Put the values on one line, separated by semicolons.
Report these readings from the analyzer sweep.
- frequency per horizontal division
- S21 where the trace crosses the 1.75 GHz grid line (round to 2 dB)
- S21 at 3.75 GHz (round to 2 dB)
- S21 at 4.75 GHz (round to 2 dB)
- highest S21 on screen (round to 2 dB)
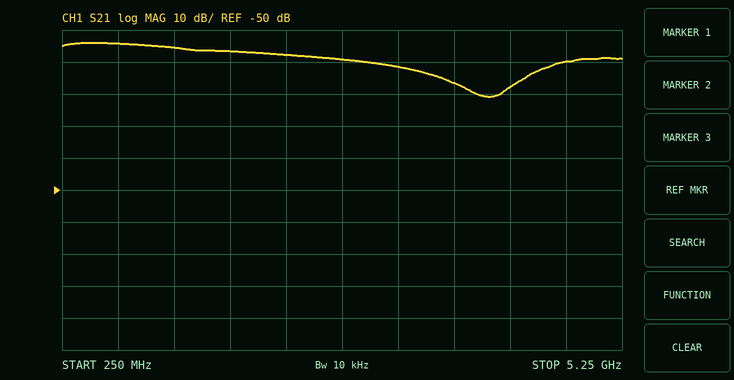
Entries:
500 MHz; -6 dB; -16 dB; -10 dB; -4 dB
